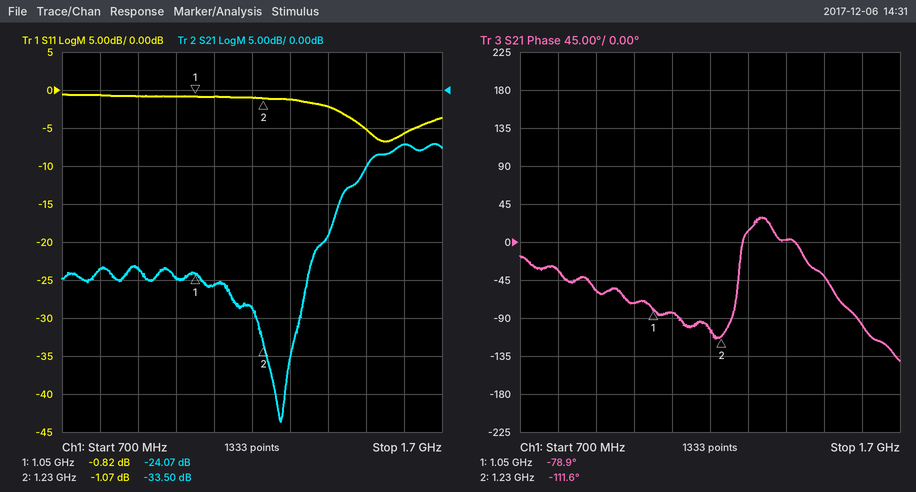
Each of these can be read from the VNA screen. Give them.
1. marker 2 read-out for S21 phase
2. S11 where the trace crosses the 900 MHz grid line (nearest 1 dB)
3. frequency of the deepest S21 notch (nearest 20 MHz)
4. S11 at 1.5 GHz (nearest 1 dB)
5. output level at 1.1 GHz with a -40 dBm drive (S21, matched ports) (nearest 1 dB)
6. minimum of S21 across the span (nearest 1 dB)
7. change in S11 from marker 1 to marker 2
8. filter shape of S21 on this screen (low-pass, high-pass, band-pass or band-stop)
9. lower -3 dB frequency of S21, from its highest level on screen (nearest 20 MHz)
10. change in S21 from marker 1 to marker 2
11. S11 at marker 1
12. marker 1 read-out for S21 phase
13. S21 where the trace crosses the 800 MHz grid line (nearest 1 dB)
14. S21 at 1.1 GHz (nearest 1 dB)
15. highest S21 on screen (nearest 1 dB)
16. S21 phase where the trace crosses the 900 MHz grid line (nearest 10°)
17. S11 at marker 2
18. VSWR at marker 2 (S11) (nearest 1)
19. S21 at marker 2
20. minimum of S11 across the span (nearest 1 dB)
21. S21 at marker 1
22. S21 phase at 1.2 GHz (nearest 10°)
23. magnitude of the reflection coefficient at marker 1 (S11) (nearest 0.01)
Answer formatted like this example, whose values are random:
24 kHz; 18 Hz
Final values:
-111.6°; -1 dB; 1.28 GHz; -5 dB; -66 dBm; -44 dB; -0.25 dB; high-pass; 1.50 GHz; -9.43 dB; -0.82 dB; -78.9°; -24 dB; -26 dB; -7 dB; -60°; -1.07 dB; 16; -33.50 dB; -7 dB; -24.07 dB; -100°; 0.91
